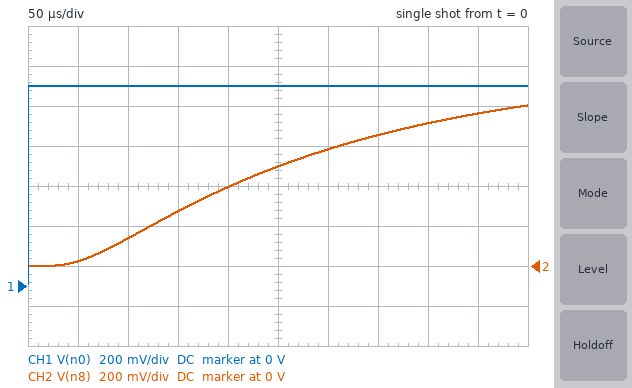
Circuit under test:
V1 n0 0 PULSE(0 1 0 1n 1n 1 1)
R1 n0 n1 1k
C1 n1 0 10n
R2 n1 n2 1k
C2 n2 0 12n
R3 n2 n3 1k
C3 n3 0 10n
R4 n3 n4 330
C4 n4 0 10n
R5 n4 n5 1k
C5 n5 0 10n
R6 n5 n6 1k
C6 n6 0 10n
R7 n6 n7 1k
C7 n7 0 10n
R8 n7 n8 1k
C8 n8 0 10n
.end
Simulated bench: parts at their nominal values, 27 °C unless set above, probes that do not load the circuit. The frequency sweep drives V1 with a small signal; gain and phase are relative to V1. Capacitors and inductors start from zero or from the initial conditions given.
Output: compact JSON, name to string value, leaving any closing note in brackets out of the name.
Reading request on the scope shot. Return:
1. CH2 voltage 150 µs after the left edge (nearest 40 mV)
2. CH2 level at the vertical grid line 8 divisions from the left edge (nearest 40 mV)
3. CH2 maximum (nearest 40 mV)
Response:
{"CH2 voltage 150 µs after the left edge": "280 mV", "CH2 level at the vertical grid line 8 divisions from the left edge": "720 mV", "CH2 maximum": "800 mV"}
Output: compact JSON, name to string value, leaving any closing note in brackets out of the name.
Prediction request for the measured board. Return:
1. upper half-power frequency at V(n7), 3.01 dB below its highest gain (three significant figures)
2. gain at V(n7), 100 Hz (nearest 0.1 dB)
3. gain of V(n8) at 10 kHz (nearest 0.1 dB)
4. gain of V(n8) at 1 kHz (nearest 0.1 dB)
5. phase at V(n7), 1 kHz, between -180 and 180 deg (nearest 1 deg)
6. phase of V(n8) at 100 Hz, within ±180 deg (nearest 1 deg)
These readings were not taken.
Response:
{"upper half-power frequency at V(n7), 3.01 dB below its highest gain": "587 Hz", "gain at V(n7), 100 Hz": "-0.1 dB", "gain of V(n8) at 10 kHz": "-35.1 dB", "gain of V(n8) at 1 kHz": "-6.0 dB", "phase at V(n7), 1 kHz, between -180 and 180 deg": "-78 deg", "phase of V(n8) at 100 Hz, within ±180 deg": "-12 deg"}
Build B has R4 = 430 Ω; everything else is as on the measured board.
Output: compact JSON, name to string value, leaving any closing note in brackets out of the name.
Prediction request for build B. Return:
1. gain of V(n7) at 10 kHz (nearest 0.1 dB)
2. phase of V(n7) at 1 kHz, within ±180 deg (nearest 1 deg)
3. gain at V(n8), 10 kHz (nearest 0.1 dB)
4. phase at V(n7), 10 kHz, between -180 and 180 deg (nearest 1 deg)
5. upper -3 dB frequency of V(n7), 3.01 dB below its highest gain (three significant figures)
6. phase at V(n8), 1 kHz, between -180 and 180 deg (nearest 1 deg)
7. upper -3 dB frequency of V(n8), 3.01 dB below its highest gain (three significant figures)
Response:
{"gain of V(n7) at 10 kHz": "-33.9 dB", "phase of V(n7) at 1 kHz, within ±180 deg": "-79 deg", "gain at V(n8), 10 kHz": "-35.3 dB", "phase at V(n7), 10 kHz, between -180 and 180 deg": "138 deg", "upper -3 dB frequency of V(n7), 3.01 dB below its highest gain": "578 Hz", "phase at V(n8), 1 kHz, between -180 and 180 deg": "-83 deg", "upper -3 dB frequency of V(n8), 3.01 dB below its highest gain": "577 Hz"}
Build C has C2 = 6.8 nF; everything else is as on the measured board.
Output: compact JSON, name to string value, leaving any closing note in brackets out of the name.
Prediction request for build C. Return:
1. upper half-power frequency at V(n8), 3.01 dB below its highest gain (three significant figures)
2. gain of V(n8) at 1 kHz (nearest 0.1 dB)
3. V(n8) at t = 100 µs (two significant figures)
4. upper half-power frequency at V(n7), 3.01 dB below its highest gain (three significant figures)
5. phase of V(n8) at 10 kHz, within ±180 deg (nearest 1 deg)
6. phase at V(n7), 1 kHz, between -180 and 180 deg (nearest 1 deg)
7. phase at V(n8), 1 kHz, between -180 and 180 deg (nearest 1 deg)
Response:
{"upper half-power frequency at V(n8), 3.01 dB below its highest gain": "599 Hz", "gain of V(n8) at 1 kHz": "-5.9 dB", "V(n8) at t = 100 µs": "150 mV", "upper half-power frequency at V(n7), 3.01 dB below its highest gain": "600 Hz", "phase of V(n8) at 10 kHz, within ±180 deg": "117 deg", "phase at V(n7), 1 kHz, between -180 and 180 deg": "-76 deg", "phase at V(n8), 1 kHz, between -180 and 180 deg": "-80 deg"}
